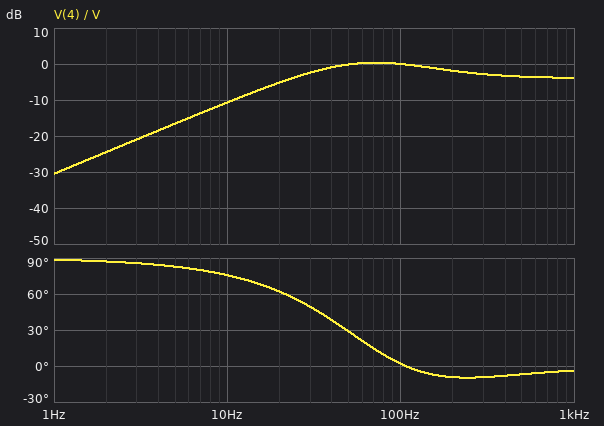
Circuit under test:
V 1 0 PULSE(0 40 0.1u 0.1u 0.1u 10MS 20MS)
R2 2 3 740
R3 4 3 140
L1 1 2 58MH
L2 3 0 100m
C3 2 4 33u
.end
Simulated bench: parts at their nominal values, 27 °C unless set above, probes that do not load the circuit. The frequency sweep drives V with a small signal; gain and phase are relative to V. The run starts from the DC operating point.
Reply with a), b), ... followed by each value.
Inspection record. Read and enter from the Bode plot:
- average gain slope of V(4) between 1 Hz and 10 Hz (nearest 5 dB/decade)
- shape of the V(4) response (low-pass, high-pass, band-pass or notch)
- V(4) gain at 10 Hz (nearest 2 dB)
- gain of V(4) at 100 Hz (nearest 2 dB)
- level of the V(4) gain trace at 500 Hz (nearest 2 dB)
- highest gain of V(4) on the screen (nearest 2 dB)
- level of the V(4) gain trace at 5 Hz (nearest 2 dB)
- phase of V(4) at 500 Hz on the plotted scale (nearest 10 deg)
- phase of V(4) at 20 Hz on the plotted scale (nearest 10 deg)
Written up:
a) 20 dB/decade
b) high-pass
c) -10 dB
d) 0 dB
e) -4 dB
f) 0 dB
g) -16 dB
h) -10 deg
i) 60 deg
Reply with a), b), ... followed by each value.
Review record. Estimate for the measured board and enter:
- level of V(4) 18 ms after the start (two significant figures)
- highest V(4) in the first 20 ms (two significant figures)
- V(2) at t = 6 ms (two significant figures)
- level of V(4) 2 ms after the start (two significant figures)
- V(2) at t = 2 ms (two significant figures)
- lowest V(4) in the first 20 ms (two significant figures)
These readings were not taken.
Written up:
a) -7.3 V
b) 31 V
c) 42 V
d) 30 V
e) 38 V
f) -29 V
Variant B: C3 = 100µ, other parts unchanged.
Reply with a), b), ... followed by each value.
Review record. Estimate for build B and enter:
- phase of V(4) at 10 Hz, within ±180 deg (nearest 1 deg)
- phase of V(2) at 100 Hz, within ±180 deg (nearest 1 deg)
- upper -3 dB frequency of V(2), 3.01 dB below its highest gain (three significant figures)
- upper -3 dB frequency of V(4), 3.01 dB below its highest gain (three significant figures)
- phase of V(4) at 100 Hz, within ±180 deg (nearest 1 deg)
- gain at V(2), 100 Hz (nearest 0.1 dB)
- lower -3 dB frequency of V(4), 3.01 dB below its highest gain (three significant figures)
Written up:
a) 49 deg
b) -13 deg
c) 236 Hz
d) 268 Hz
e) -8 deg
f) -1.2 dB
g) 10.7 Hz
